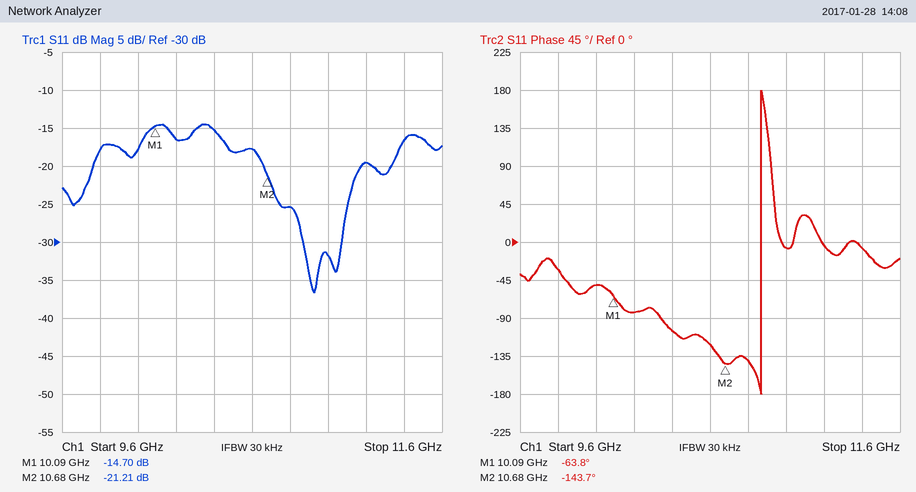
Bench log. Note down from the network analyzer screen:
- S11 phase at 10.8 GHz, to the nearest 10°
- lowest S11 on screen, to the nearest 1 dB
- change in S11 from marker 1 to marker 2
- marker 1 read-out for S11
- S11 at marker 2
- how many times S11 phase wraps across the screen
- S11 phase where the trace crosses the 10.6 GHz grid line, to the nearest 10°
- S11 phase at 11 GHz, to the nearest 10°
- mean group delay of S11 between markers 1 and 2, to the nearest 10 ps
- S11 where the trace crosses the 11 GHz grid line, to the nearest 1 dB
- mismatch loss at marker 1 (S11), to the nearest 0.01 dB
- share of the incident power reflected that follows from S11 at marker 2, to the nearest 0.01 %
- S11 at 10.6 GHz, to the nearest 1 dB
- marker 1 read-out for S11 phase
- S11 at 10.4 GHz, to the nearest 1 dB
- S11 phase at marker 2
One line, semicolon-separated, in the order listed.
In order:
-140°; -37 dB; -6.51 dB; -14.70 dB; -21.21 dB; 1; -120°; -10°; 380 ps; -32 dB; 0.15 dB; 0.76 %; -18 dB; -63.8°; -15 dB; -143.7°
